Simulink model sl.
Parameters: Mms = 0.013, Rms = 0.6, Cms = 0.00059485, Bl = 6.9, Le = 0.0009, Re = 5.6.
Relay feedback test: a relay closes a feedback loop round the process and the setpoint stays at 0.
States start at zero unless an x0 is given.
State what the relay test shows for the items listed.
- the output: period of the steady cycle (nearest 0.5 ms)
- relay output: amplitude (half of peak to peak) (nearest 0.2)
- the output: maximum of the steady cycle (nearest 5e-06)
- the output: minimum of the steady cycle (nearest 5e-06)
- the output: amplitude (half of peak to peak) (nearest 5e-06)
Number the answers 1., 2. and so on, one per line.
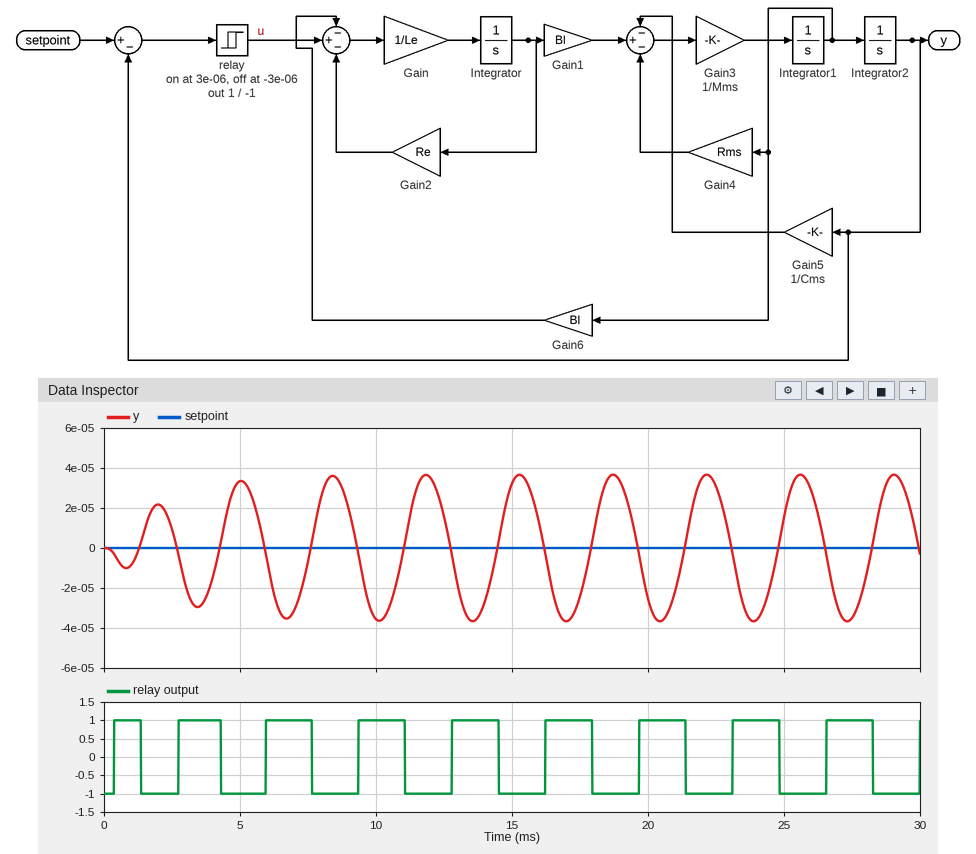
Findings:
1. 3.5 ms
2. 1.0
3. 0.000035
4. -0.000035
5. 0.000035
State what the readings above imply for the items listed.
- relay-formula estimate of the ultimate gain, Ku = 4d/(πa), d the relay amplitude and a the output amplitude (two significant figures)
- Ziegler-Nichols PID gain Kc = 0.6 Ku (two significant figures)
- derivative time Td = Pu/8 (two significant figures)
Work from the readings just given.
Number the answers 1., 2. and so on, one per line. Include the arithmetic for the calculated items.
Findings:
1. 4 × 1 / (π × 3.5e-05) = 36000
2. 0.6 × 36000 = 22000
3. 3.5 / 8 = 0.44 ms
